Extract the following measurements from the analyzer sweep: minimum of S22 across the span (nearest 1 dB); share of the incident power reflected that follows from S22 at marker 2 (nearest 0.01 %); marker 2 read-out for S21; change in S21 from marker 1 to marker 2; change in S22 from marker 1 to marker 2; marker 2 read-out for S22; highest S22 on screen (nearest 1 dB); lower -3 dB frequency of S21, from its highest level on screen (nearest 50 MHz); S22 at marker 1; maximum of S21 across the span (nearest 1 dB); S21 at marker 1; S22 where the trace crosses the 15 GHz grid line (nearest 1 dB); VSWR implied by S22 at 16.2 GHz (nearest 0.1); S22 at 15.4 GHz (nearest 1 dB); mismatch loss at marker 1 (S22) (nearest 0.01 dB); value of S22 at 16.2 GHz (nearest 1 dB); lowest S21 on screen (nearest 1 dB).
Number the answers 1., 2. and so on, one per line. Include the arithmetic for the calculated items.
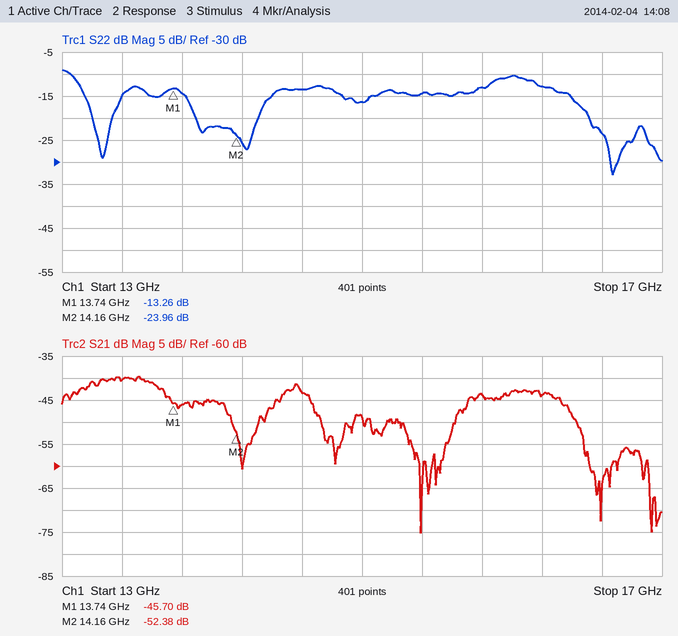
1. -33 dB
2. 10^(-23.96/10) ≈ 0.40 %
3. -52.38 dB
4. -52.38 − (-45.7) = -6.68 dB
5. -23.96 − (-13.26) = -10.70 dB
6. -23.96 dB
7. -9 dB
8. 13.10 GHz
9. -13.26 dB
10. -40 dB
11. -45.70 dB
12. -16 dB
13. |Γ| = 10^(-13/20) = 0.2239; VSWR = (1 + 0.2239)/(1 − 0.2239) ≈ 1.6
14. -14 dB
15. −10 log10(1 − 10^(-13.26/10)) ≈ 0.21 dB
16. -13 dB
17. -75 dB
